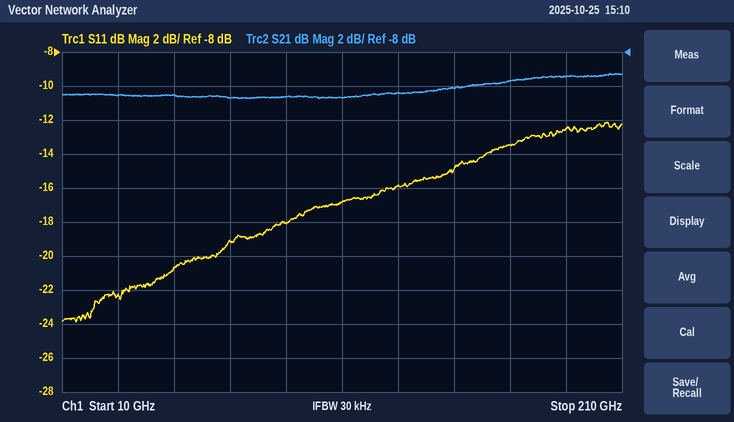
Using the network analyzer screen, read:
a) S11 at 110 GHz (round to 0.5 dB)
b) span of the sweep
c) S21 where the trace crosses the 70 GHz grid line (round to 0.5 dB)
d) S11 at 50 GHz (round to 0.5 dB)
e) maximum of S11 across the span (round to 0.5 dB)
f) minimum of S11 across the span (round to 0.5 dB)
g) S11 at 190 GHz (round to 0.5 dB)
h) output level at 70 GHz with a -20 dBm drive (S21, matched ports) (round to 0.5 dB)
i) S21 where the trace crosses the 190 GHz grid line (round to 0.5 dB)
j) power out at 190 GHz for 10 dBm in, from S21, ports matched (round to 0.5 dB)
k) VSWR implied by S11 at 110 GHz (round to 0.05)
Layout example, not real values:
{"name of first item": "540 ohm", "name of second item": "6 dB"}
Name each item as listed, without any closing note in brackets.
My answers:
{"S11 at 110 GHz": "-17.0 dB", "span of the sweep": "200 GHz", "S21 where the trace crosses the 70 GHz grid line": "-10.5 dB", "S11 at 50 GHz": "-20.5 dB", "maximum of S11 across the span": "-12.0 dB", "minimum of S11 across the span": "-24.0 dB", "S11 at 190 GHz": "-12.5 dB", "output level at 70 GHz with a -20 dBm drive (S21, matched ports)": "-30.5 dBm", "S21 where the trace crosses the 190 GHz grid line": "-9.5 dB", "power out at 190 GHz for 10 dBm in, from S21, ports matched": "0.5 dBm", "VSWR implied by S11 at 110 GHz": "1.35"}
